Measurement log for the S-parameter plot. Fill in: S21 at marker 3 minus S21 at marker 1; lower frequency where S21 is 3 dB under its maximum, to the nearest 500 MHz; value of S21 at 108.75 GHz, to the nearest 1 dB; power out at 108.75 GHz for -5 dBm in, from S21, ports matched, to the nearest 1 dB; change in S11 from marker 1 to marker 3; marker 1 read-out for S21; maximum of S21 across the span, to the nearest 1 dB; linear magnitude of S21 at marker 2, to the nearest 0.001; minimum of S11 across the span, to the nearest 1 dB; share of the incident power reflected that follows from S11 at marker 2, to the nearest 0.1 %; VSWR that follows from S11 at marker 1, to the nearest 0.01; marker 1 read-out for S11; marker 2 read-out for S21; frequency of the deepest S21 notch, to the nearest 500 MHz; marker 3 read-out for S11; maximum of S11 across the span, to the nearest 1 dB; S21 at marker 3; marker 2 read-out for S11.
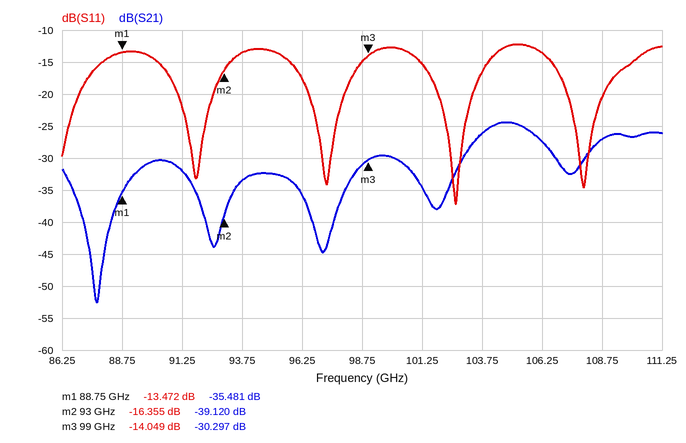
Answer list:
5.184 dB
103.5 GHz
-27 dB
-32 dBm
-0.577 dB
-35.481 dB
-24 dB
0.011
-37 dB
2.3 %
1.54
-13.472 dB
-39.120 dB
87.5 GHz
-14.049 dB
-12 dB
-30.297 dB
-16.355 dB
